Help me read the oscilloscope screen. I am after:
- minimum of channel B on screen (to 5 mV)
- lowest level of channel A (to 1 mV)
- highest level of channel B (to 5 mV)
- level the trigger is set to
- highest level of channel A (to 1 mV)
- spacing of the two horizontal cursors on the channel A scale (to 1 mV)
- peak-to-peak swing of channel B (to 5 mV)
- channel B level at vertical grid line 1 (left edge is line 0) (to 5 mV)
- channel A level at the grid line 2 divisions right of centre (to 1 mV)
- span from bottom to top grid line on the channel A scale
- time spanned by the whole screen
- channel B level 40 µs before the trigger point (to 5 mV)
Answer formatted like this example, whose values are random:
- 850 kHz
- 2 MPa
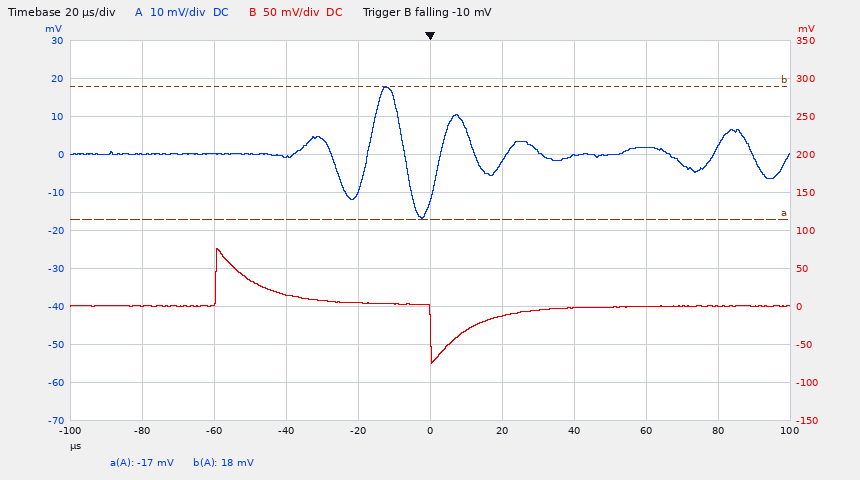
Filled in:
- -75 mV
- -17 mV
- 75 mV
- -10 mV
- 18 mV
- 35 mV
- 150 mV
- 0 mV
- 0 mV
- 100 mV
- 200 µs
- 15 mV
